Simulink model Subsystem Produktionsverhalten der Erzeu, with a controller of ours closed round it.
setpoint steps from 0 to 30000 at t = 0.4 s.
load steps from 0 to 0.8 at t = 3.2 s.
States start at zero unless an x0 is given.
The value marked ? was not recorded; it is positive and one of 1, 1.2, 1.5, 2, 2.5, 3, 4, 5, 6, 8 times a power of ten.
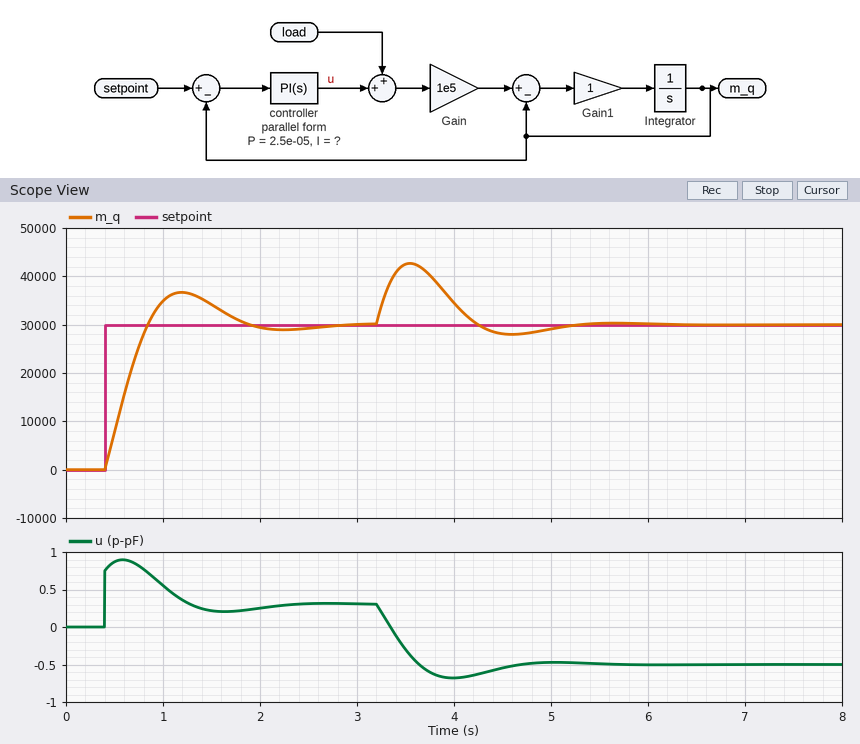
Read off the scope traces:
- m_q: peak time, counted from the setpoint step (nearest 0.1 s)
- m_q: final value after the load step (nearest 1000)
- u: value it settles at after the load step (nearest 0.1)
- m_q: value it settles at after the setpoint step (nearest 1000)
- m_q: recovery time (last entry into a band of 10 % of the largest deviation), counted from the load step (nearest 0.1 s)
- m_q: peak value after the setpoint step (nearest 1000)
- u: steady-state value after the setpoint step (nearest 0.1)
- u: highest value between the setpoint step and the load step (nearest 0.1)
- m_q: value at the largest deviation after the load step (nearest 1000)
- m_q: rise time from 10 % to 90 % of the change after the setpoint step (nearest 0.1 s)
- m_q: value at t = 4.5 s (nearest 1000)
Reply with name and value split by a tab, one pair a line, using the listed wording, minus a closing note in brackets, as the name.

m_q: peak time, counted from the setpoint step	0.8 s
m_q: final value after the load step	30000
u: value it settles at after the load step	-0.5
m_q: value it settles at after the setpoint step	30000
m_q: recovery time (last entry into a band of 10 % of the largest deviation), counted from the load step	1.7 s
m_q: peak value after the setpoint step	37000
u: steady-state value after the setpoint step	0.3
u: highest value between the setpoint step and the load step	0.9
m_q: value at the largest deviation after the load step	43000
m_q: rise time from 10 % to 90 % of the change after the setpoint step	0.3 s
m_q: value at t = 4.5 s	28000
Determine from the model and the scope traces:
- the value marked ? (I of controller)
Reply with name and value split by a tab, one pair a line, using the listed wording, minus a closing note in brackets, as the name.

the value marked ?	0.00012
